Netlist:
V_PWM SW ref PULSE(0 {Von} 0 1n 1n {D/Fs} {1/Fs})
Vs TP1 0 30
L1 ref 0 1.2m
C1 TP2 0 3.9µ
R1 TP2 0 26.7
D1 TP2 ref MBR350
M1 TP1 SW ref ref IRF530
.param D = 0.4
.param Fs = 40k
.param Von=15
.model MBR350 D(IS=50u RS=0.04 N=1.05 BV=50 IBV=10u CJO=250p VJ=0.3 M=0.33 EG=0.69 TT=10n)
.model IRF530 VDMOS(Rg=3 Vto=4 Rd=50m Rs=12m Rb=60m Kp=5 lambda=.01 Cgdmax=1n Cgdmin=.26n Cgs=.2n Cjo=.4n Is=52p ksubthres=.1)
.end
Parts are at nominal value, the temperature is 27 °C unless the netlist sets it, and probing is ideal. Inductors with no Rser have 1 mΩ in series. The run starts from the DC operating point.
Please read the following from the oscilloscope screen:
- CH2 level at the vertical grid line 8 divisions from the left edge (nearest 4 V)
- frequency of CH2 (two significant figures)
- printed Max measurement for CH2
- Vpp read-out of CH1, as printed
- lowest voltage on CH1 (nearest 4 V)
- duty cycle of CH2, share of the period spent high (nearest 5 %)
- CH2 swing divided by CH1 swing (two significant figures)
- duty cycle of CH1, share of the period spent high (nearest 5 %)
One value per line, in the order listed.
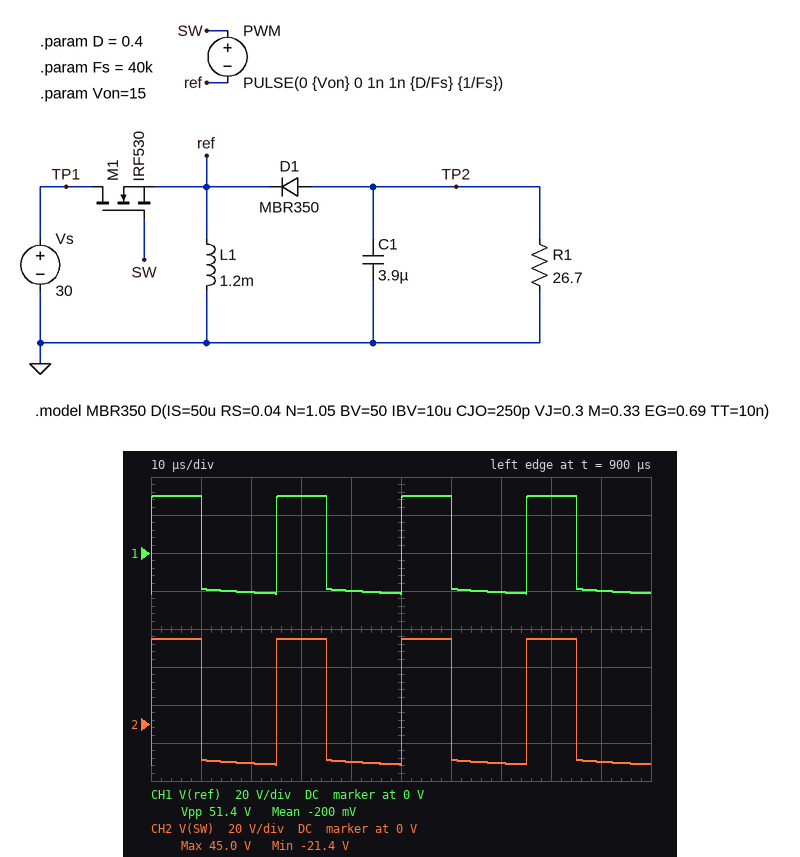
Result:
44 V
40 kHz
45.0 V
51.4 V
-20 V
40 %
1.3
40 %
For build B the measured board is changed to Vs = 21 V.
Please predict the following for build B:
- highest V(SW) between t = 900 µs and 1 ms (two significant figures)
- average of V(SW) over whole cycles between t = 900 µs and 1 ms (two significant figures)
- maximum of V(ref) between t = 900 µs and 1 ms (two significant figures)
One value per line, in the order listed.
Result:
36 V
6.1 V
21 V
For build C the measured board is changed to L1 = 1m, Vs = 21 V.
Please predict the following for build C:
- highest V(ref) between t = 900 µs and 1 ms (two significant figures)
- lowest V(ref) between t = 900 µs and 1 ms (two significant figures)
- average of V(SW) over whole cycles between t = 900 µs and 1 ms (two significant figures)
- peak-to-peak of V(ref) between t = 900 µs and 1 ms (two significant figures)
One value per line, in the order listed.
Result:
21 V
-15 V
6.0 V
36 V
